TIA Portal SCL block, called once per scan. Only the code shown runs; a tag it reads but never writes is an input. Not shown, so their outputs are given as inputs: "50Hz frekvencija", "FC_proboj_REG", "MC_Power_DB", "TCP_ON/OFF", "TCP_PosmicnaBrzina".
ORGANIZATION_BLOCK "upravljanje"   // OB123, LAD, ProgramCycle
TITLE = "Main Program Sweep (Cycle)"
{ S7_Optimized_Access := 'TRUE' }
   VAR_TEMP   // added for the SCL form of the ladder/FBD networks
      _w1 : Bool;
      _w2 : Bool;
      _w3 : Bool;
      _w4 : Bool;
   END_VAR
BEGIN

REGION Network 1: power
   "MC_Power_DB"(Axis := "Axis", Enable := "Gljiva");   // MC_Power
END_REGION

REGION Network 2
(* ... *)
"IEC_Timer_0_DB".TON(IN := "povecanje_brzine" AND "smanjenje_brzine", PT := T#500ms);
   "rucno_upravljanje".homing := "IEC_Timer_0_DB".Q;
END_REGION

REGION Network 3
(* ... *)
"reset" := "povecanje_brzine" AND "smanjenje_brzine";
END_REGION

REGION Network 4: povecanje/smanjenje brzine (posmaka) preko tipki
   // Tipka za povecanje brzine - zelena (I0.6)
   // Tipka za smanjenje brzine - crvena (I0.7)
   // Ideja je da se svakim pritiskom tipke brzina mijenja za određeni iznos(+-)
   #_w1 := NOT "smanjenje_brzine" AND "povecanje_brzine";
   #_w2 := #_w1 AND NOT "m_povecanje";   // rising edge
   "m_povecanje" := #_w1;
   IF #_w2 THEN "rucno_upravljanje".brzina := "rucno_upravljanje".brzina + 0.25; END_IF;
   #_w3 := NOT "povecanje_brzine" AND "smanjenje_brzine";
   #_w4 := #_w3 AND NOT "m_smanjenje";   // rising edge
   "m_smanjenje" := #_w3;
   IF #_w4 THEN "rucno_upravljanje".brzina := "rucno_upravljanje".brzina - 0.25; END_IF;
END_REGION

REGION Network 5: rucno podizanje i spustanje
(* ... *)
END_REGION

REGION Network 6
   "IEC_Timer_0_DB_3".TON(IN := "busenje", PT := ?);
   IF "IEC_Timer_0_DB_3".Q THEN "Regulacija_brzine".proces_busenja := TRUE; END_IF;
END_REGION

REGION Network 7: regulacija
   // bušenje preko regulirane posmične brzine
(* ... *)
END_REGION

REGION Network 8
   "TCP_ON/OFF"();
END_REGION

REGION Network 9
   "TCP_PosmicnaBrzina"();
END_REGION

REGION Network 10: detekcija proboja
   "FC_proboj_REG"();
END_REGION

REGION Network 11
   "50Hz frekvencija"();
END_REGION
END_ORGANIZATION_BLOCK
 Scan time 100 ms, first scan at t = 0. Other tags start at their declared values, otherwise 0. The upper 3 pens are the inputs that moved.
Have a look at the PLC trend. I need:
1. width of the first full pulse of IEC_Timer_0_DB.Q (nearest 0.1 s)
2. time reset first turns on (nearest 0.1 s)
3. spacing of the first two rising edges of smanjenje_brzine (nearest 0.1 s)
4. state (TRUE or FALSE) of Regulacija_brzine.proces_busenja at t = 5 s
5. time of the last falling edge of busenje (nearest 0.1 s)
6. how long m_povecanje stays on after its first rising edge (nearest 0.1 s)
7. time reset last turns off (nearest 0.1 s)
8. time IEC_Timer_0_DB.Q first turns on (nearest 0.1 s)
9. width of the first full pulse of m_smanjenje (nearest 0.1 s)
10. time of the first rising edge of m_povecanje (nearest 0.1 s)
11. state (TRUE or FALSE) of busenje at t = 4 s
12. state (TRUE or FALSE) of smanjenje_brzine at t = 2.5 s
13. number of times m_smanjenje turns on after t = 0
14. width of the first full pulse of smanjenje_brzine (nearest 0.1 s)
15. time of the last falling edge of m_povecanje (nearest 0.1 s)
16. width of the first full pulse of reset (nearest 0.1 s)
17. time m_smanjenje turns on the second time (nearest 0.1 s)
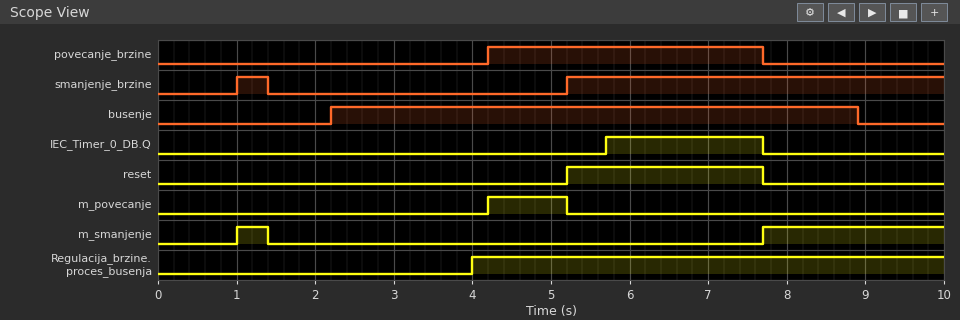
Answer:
2.0 s
5.2 s
4.2 s
TRUE
8.9 s
1.0 s
7.7 s
5.7 s
0.4 s
4.2 s
TRUE
FALSE
2
0.4 s
5.2 s
2.5 s
7.7 s
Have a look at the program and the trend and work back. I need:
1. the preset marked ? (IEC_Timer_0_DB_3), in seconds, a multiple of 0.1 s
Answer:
1.8 s
